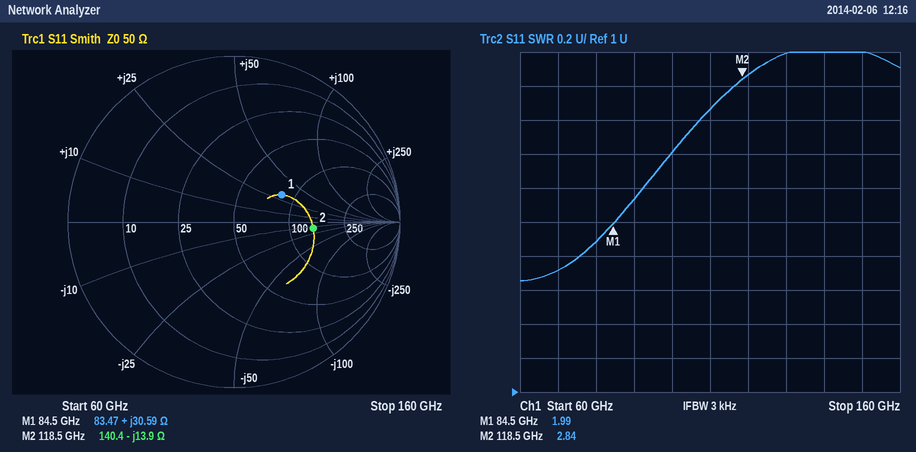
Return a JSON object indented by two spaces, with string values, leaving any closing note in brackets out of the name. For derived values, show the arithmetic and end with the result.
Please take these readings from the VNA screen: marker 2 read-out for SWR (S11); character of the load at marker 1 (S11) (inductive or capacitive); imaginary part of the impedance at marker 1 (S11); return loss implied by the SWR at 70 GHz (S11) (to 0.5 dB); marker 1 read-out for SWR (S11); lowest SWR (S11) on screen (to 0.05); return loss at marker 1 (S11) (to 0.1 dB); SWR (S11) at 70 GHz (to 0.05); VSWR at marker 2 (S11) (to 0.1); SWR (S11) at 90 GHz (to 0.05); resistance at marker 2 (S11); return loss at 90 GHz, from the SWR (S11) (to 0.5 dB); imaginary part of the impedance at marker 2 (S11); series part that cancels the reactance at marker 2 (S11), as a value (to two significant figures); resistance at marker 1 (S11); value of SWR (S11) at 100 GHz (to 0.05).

{
  "marker 2 read-out for SWR": "2.84",
  "character of the load at marker 1 (S11)": "inductive",
  "imaginary part of the impedance at marker 1": "+30.59 Ω",
  "return loss implied by the SWR at 70 GHz (S11)": "−20 log10((1.7 − 1)/(1.7 + 1)) ≈ 11.7 dB, so 11.5 dB to the nearest 0.5 dB",
  "marker 1 read-out for SWR": "1.99",
  "lowest SWR (S11) on screen": "1.65",
  "return loss at marker 1 (S11)": "9.6 dB",
  "SWR (S11) at 70 GHz": "1.70",
  "VSWR at marker 2 (S11)": "2.8",
  "SWR (S11) at 90 GHz": "2.15",
  "resistance at marker 2": "140.4 Ω",
  "return loss at 90 GHz, from the SWR (S11)": "−20 log10((2.15 − 1)/(2.15 + 1)) ≈ 8.75 dB, so 9.0 dB to the nearest 0.5 dB",
  "imaginary part of the impedance at marker 2": "-13.9 Ω",
  "series part that cancels the reactance at marker 2 (S11), as a value": "L = 13.9 Ω/(2π × 118.5 GHz) ≈ 19 pH",
  "resistance at marker 1": "83.47 Ω",
  "value of SWR (S11) at 100 GHz": "2.40"
}
